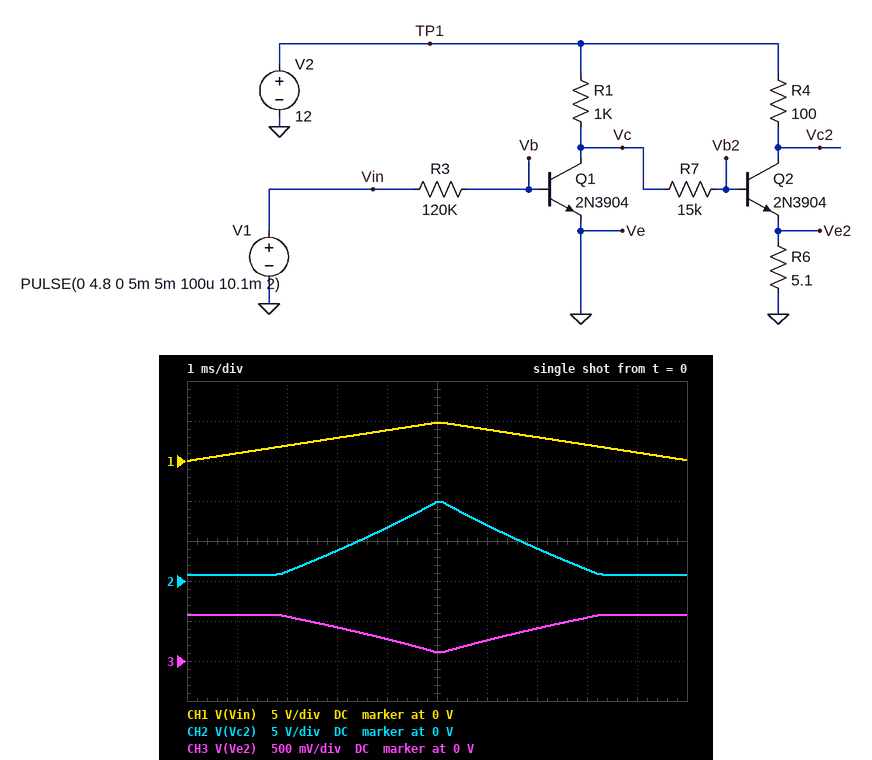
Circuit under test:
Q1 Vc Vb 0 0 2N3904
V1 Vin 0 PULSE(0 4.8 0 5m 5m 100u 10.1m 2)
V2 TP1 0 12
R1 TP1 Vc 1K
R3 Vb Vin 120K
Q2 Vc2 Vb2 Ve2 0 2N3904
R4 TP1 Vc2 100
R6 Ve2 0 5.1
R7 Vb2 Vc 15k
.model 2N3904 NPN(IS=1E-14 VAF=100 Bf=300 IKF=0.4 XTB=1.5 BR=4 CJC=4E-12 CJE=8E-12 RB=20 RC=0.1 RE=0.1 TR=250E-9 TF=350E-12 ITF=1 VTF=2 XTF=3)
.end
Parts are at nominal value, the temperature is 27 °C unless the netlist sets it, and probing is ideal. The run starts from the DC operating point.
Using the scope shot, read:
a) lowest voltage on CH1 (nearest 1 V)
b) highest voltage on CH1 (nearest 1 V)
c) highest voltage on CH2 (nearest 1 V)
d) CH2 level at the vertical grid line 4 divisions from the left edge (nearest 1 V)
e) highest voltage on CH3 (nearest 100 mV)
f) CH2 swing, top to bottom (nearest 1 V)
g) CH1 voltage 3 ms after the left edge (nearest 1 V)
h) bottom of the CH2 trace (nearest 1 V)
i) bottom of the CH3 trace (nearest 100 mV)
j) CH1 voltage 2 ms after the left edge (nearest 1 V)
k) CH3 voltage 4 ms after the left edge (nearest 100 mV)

0 V
5 V
10 V
7 V
600 mV
9 V
3 V
1 V
100 mV
2 V
300 mV
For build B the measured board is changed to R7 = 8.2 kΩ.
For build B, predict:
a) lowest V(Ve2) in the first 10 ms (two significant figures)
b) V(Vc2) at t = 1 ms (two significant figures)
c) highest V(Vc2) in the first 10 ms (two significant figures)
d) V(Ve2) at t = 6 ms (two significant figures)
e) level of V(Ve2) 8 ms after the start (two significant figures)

170 mV
710 mV
8.7 V
390 mV
580 mV
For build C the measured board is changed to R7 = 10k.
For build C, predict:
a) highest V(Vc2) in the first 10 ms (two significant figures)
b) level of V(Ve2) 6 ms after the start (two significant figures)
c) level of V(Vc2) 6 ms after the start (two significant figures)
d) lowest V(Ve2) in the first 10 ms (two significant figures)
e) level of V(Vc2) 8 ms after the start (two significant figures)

9.1 V
340 mV
5.3 V
150 mV
740 mV
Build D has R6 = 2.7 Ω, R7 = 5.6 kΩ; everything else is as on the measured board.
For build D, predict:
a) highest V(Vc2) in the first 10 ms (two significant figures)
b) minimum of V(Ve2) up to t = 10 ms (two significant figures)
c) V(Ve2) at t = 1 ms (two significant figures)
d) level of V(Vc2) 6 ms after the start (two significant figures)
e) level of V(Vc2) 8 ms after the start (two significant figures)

7.4 V
120 mV
320 mV
1.8 V
450 mV
